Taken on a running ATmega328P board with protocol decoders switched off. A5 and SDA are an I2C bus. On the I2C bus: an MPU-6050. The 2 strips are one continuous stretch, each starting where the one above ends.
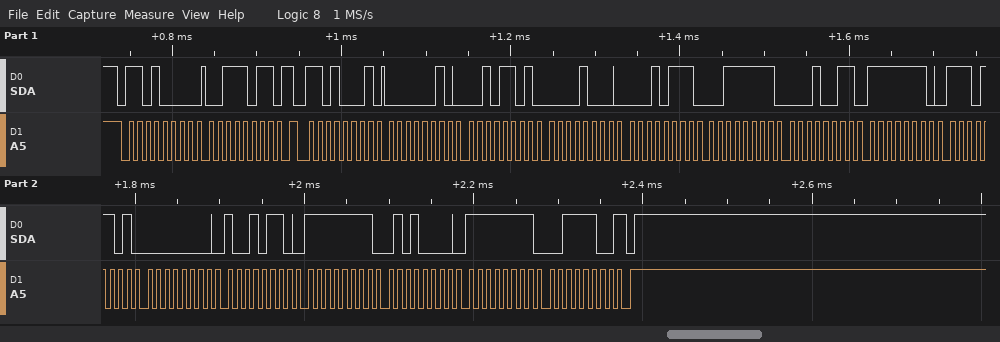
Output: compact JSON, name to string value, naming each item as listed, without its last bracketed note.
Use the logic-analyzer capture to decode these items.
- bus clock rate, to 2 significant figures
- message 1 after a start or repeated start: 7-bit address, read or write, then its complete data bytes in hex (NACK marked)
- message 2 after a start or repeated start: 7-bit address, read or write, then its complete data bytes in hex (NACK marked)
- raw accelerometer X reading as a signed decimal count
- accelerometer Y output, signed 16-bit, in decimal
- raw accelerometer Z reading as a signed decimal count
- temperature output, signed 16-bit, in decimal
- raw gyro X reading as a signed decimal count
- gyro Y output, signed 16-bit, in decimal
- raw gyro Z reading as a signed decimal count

{"bus clock rate, to 2 significant figures": "100 kHz", "message 1 after a start or repeated start: 7-bit address, read or write, then its complete data bytes in hex": "0x68 write: 3B", "message 2 after a start or repeated start: 7-bit address, read or write, then its complete data bytes in hex": "0x68 read: 02 2D 08 17 3F 13 FE ED 00 96 FF 50 FF 3C NACK", "raw accelerometer X reading as a signed decimal count": "557", "accelerometer Y output, signed 16-bit, in decimal": "2071", "raw accelerometer Z reading as a signed decimal count": "16147", "temperature output, signed 16-bit, in decimal": "-275", "raw gyro X reading as a signed decimal count": "150", "gyro Y output, signed 16-bit, in decimal": "-176", "raw gyro Z reading as a signed decimal count": "-196"}
